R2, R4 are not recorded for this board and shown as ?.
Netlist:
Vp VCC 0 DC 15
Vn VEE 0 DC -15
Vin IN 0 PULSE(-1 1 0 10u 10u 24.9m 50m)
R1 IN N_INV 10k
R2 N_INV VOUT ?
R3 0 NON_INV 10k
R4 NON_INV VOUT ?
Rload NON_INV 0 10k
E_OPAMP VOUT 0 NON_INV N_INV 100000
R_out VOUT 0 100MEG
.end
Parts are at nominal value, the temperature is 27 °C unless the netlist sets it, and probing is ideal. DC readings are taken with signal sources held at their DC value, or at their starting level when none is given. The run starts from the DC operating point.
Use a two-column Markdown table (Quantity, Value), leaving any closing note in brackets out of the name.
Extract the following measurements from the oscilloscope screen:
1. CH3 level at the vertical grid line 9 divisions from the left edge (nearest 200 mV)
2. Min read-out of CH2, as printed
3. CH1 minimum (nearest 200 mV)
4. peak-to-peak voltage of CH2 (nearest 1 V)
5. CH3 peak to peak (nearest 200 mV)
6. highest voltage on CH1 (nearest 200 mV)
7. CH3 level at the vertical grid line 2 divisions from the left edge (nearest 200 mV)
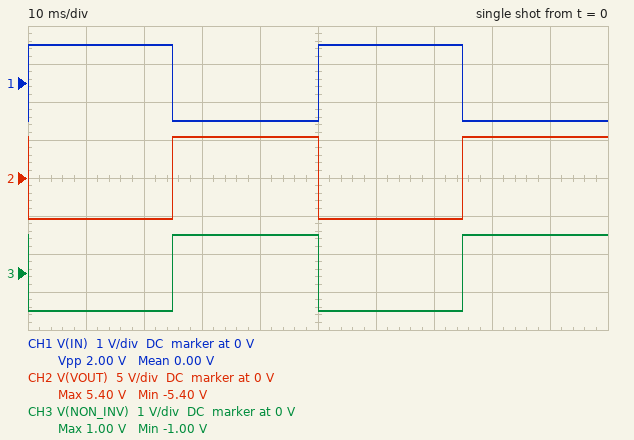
| Quantity | Value |
|---|---|
| CH3 level at the vertical grid line 9 divisions from the left edge | 1.0 V |
| Min read-out of CH2, as printed | -5.40 V |
| CH1 minimum | -1.0 V |
| peak-to-peak voltage of CH2 | 11 V |
| CH3 peak to peak | 2.0 V |
| highest voltage on CH1 | 1.0 V |
| CH3 level at the vertical grid line 2 divisions from the left edge | -1.0 V |
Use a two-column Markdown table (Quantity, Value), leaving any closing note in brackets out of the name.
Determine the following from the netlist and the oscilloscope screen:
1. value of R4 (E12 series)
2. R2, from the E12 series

| Quantity | Value |
|---|---|
| value of R4 | 22 kΩ |
| R2, from the E12 series | 22 kΩ |
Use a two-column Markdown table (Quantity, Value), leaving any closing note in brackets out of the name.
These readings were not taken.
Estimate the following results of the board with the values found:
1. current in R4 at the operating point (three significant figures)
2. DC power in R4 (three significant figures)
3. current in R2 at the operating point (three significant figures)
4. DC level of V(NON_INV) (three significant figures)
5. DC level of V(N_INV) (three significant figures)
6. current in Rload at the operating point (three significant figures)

| Quantity | Value |
|---|---|
| current in R4 at the operating point | 200 µA |
| DC power in R4 | 880 µW |
| current in R2 at the operating point | 200 µA |
| DC level of V(NON_INV) | 1.00 V |
| DC level of V(N_INV) | 1.00 V |
| current in Rload at the operating point | 100 µA |
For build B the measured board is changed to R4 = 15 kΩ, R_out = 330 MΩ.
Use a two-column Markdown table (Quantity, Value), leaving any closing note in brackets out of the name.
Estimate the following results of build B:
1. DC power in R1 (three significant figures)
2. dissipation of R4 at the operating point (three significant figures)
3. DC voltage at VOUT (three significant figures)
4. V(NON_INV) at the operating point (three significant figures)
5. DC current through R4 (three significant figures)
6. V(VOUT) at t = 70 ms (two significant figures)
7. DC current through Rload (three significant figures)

| Quantity | Value |
|---|---|
| DC power in R1 | 1.41 mW |
| dissipation of R4 at the operating point | 4.54 mW |
| DC voltage at VOUT | 11.0 V |
| V(NON_INV) at the operating point | 2.75 V |
| DC current through R4 | 550 µA |
| V(VOUT) at t = 70 ms | -11 V |
| DC current through Rload | 275 µA |
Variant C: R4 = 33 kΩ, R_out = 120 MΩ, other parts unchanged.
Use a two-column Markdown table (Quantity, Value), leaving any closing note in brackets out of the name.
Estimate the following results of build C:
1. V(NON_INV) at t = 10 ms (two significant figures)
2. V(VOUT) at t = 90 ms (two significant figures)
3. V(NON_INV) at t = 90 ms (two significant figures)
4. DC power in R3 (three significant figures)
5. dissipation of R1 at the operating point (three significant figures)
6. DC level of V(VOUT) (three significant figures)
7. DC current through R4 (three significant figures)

| Quantity | Value |
|---|---|
| V(NON_INV) at t = 10 ms | -500 mV |
| V(VOUT) at t = 90 ms | 3.8 V |
| V(NON_INV) at t = 90 ms | 500 mV |
| DC power in R3 | 25.0 µW |
| dissipation of R1 at the operating point | 225 µW |
| DC level of V(VOUT) | 3.80 V |
| DC current through R4 | 100 µA |
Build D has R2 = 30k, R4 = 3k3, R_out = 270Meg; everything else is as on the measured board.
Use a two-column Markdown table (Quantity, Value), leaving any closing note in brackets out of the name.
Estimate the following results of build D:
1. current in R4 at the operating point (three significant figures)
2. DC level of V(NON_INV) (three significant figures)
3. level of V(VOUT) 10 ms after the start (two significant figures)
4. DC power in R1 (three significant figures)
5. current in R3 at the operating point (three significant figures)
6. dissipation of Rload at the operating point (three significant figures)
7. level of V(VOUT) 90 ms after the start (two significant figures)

| Quantity | Value |
|---|---|
| current in R4 at the operating point | 256 µA |
| DC level of V(NON_INV) | -1.28 V |
| level of V(VOUT) 10 ms after the start | 2.1 V |
| DC power in R1 | 7.96 µW |
| current in R3 at the operating point | 128 µA |
| dissipation of Rload at the operating point | 164 µW |
| level of V(VOUT) 90 ms after the start | -2.1 V |
